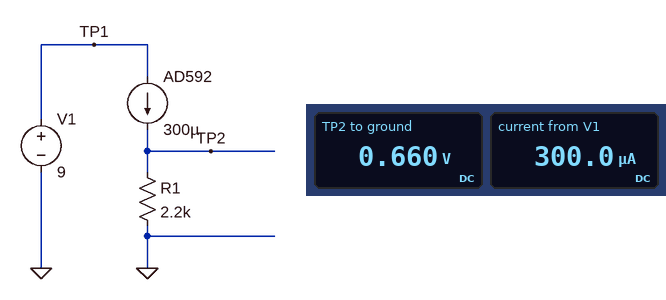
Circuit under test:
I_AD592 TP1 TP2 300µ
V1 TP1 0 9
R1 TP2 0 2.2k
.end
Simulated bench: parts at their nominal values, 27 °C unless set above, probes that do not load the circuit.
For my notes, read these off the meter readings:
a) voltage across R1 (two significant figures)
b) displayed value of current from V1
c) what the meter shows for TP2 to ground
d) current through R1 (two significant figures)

660 mV
300.0 µA
0.660 V
300 µA
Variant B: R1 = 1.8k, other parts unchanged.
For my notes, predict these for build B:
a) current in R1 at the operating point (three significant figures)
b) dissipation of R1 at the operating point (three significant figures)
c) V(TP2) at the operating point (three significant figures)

300 µA
162 µW
540 mV
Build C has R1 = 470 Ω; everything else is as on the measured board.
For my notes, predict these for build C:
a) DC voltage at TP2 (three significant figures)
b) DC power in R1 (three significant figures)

141 mV
42.3 µW
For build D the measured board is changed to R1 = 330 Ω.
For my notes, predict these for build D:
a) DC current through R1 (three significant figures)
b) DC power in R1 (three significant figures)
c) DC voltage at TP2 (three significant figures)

300 µA
29.7 µW
99.0 mV
